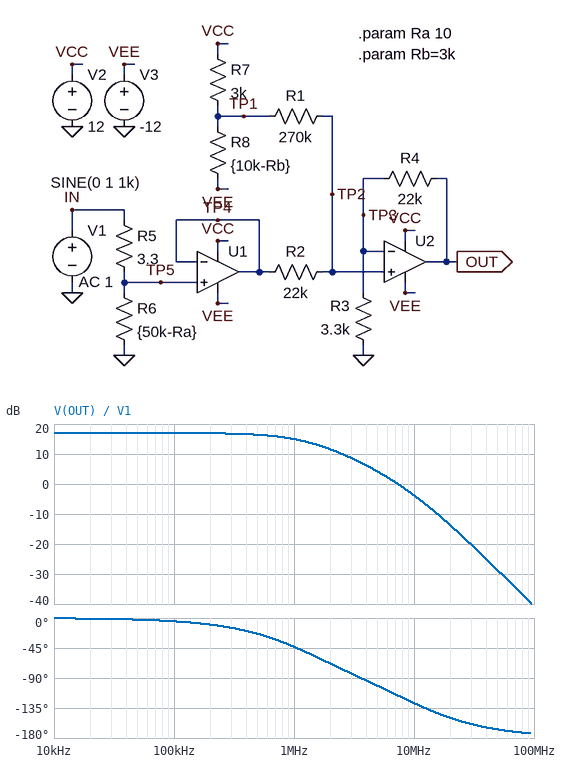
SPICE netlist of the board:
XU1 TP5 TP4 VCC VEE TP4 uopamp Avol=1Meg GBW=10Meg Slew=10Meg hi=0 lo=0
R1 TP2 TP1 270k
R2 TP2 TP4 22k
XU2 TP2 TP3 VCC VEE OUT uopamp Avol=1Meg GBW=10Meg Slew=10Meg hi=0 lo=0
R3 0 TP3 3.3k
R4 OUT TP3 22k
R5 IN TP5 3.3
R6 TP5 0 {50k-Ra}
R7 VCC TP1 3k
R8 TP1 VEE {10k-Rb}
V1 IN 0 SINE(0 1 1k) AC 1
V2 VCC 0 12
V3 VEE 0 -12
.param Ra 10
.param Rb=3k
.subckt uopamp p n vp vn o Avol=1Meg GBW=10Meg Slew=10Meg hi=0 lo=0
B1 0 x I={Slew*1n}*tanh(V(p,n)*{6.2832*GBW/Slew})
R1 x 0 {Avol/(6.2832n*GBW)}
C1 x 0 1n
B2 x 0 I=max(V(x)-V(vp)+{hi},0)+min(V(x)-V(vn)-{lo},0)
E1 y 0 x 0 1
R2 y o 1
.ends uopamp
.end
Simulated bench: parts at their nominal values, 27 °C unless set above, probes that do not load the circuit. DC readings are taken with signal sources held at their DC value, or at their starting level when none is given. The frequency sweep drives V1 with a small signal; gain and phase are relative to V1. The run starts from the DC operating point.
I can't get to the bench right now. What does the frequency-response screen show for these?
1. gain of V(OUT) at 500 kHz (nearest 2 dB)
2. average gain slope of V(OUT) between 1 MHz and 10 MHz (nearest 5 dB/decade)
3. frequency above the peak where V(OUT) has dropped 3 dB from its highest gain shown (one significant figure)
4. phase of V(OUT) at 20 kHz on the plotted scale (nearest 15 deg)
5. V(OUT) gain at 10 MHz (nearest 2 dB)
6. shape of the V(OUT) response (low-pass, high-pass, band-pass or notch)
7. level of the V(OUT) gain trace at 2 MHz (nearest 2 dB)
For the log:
16 dB
-20 dB/decade
1 MHz
0 deg
-4 dB
low-pass
12 dB
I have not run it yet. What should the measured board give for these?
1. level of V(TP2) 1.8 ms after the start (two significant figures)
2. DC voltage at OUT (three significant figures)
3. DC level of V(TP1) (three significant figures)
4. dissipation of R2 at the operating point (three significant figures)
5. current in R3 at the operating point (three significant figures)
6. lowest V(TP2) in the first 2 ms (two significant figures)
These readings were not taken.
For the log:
-520 mV
2.75 V
4.77 V
5.86 µW
109 µA
-570 mV
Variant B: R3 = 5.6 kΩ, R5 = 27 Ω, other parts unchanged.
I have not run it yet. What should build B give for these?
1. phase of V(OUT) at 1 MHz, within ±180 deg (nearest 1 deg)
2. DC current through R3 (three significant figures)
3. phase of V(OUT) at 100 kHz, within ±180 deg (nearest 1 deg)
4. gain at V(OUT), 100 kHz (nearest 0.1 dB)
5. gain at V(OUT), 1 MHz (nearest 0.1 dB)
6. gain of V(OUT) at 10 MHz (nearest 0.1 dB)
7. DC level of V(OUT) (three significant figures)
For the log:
-32 deg
64.1 µA
-3 deg
13.2 dB
12.2 dB
-3.9 dB
1.77 V
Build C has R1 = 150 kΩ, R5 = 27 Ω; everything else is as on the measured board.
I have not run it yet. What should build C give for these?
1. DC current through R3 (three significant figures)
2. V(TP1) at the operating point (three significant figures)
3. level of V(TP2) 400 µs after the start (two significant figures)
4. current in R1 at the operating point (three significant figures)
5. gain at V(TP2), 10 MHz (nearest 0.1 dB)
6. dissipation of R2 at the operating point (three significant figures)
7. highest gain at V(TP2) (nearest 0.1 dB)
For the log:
184 µA
4.74 V
1.1 V
27.6 µA
-4.2 dB
16.7 µW
-1.2 dB
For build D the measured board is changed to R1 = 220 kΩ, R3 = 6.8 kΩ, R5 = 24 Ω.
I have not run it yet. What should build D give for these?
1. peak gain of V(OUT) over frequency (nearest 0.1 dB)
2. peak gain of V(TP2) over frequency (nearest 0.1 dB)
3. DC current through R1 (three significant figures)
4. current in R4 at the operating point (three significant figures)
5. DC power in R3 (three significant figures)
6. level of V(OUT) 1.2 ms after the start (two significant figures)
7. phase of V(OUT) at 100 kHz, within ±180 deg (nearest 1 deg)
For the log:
11.7 dB
-0.8 dB
19.7 µA
63.6 µA
27.5 µW
5.5 V
-3 deg
